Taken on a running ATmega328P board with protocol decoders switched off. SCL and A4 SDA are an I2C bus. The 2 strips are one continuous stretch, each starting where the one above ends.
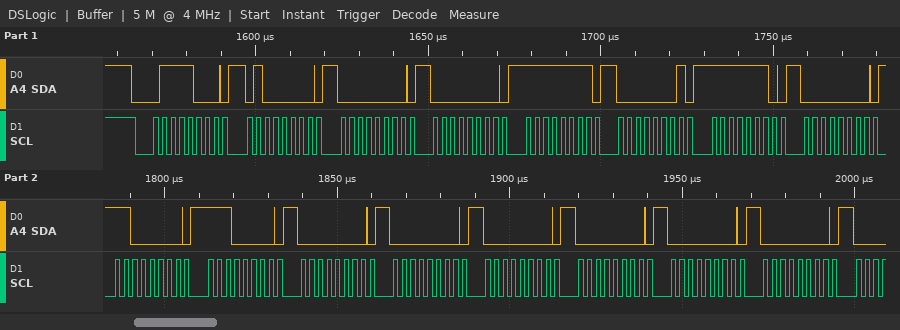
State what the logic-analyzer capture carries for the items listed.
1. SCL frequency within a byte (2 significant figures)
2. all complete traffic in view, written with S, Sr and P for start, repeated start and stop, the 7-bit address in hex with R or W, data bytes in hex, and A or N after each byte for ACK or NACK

400 kHz
S 3CW A 40 A 00 A 00 A FF A 01 A FE A 00 A C0 A E0 A 00 A 00 A 00 A 00 A 00 A 00 A
